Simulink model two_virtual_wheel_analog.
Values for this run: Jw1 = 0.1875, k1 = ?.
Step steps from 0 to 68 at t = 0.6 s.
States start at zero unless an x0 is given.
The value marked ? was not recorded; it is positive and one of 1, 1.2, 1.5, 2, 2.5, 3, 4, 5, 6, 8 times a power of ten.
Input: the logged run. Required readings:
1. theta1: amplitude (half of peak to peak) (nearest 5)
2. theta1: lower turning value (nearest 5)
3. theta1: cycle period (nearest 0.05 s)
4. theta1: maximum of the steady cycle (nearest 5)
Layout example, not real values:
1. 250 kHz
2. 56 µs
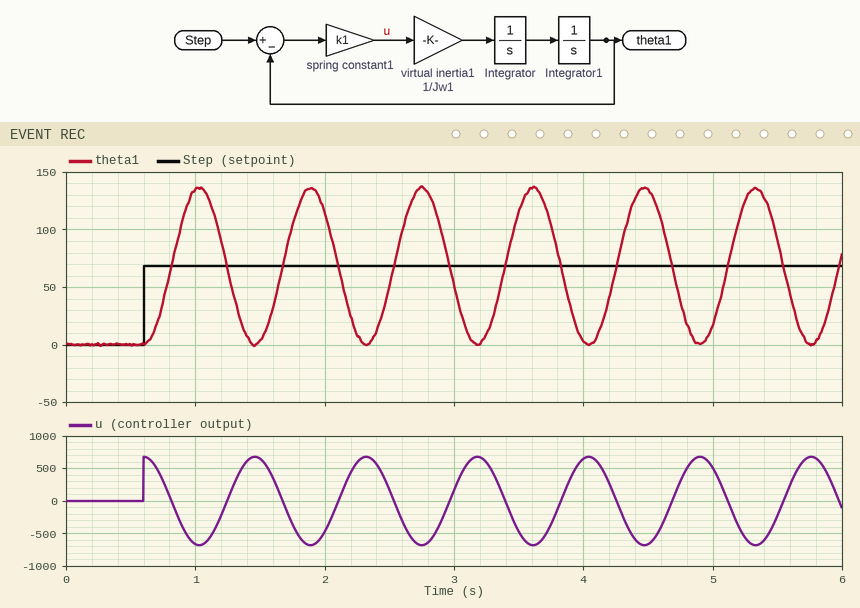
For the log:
1. 70
2. 0
3. 0.85 s
4. 135
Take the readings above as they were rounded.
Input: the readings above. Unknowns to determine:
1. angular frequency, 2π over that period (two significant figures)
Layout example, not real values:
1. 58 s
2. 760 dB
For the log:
1. 7.4 rad/s
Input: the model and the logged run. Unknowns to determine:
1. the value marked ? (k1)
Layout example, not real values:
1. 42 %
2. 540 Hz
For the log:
1. 10
